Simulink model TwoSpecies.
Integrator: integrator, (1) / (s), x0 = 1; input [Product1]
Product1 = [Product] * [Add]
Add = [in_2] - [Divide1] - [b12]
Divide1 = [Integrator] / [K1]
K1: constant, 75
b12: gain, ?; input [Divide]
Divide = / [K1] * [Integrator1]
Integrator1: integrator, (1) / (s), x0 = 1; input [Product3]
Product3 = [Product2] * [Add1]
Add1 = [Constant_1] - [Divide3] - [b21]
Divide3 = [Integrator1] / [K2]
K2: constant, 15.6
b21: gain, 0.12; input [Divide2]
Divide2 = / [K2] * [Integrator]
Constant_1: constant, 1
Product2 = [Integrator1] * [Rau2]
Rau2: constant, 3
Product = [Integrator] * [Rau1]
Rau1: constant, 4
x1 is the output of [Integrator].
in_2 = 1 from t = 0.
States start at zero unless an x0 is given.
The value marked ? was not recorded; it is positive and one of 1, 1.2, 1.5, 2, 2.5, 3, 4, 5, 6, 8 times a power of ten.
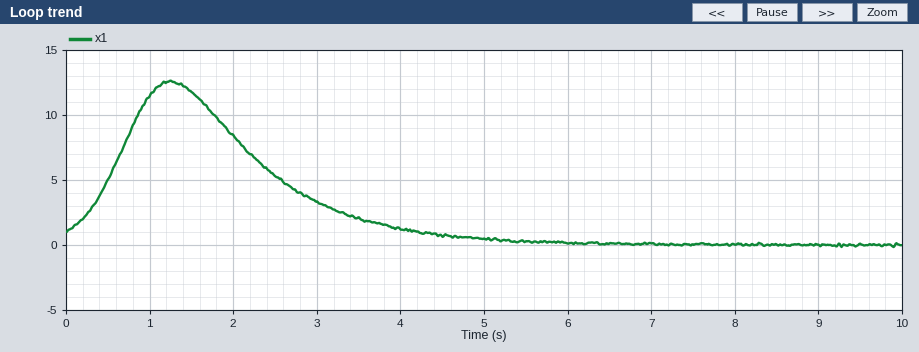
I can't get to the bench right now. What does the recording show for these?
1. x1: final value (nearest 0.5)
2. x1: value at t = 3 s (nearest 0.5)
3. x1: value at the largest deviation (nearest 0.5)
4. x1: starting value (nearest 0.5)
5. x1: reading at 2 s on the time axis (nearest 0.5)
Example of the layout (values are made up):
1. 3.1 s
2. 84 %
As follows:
1. 0.0
2. 3.5
3. 12.5
4. 1.0
5. 8.5
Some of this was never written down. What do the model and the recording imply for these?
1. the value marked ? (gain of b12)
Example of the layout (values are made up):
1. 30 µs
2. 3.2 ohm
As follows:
1. 6
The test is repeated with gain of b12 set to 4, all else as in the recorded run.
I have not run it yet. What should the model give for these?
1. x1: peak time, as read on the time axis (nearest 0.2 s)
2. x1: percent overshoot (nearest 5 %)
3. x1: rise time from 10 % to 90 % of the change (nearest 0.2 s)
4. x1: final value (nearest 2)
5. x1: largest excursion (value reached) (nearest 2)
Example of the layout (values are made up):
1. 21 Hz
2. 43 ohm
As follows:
1. 2.2 s
2. 10 %
3. 1.0 s
4. 24
5. 26
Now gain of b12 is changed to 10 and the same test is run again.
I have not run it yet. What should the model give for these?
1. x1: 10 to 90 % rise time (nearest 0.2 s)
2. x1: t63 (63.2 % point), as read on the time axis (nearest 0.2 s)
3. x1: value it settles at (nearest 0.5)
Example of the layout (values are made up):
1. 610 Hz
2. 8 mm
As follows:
1. 0.6 s
2. 2.0 s
3. 0.0
